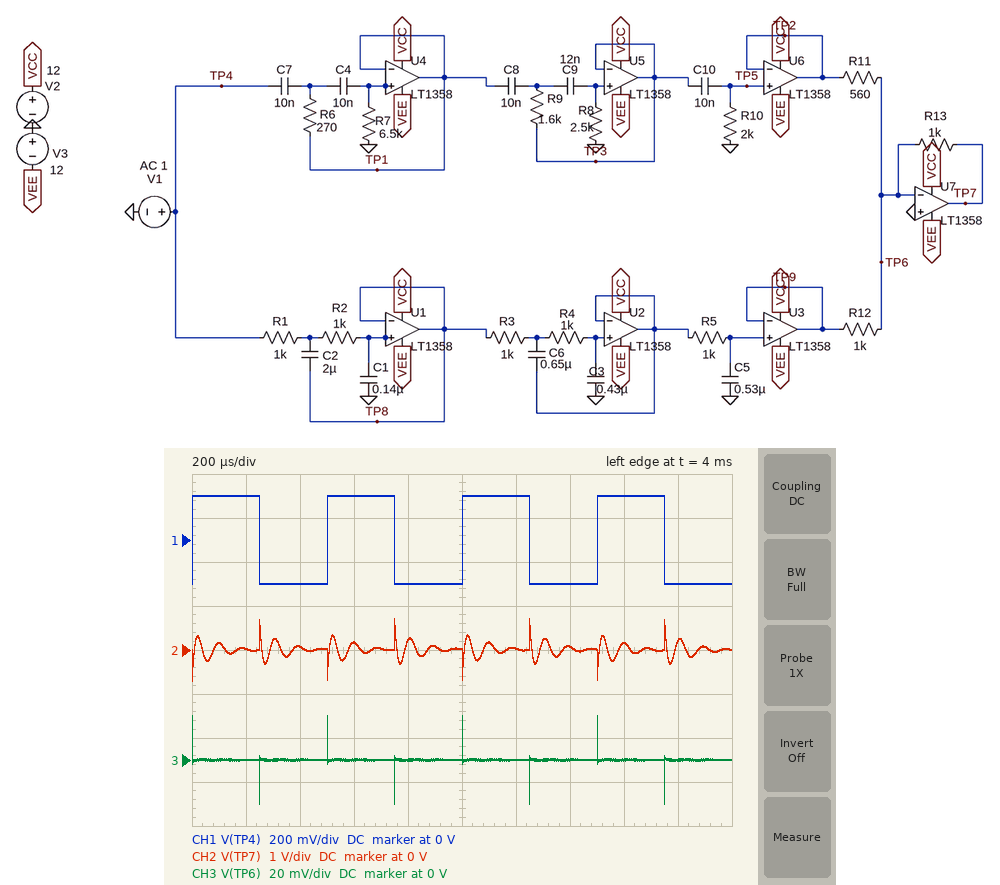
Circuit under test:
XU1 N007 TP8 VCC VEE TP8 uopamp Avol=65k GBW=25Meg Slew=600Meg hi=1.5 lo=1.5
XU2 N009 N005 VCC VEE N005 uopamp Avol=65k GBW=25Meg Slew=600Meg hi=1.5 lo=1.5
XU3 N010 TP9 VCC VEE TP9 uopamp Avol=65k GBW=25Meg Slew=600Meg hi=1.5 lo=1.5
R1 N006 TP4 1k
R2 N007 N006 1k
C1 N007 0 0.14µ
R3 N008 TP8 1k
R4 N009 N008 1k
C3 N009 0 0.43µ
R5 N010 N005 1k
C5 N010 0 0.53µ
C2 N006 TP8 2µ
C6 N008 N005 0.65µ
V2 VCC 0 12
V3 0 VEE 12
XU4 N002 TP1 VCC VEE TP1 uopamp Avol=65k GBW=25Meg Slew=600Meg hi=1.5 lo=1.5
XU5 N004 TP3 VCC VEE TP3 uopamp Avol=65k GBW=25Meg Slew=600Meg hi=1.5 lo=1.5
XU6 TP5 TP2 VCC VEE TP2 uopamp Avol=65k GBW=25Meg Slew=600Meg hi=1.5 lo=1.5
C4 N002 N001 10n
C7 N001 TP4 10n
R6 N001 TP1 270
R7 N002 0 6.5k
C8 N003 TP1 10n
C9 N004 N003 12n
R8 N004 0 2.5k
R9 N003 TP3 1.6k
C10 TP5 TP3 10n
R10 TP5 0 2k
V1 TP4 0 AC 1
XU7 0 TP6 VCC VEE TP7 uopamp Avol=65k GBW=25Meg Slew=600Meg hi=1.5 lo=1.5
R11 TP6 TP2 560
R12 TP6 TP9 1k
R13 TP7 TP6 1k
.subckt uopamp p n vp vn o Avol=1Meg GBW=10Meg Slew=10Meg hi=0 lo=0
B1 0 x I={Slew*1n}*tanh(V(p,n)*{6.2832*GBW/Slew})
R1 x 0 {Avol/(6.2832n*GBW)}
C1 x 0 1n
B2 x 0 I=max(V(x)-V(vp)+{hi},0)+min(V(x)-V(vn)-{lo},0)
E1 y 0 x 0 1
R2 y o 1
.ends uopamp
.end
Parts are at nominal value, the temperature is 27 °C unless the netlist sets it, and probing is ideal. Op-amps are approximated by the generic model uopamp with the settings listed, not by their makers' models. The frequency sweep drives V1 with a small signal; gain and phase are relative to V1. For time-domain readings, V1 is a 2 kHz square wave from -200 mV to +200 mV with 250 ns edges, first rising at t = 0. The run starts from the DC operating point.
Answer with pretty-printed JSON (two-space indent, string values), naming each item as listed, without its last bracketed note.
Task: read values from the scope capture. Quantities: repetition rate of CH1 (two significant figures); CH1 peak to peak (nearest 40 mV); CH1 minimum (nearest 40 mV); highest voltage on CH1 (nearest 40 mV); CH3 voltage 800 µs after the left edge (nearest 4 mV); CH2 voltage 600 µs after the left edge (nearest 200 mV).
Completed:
{
  "repetition rate of CH1": "2.0 kHz",
  "CH1 peak to peak": "400 mV",
  "CH1 minimum": "-200 mV",
  "highest voltage on CH1": "200 mV",
  "CH3 voltage 800 µs after the left edge": "0 V",
  "CH2 voltage 600 µs after the left edge": "200 mV"
}
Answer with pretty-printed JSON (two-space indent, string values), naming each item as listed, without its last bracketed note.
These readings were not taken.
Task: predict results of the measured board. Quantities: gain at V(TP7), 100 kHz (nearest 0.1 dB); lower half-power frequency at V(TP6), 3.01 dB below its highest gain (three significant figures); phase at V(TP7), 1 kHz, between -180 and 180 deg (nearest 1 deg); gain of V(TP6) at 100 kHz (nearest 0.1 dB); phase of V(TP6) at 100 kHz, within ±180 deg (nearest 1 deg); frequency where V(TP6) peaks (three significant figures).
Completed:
{
  "gain at V(TP7), 100 kHz": "5.1 dB",
  "lower half-power frequency at V(TP6), 3.01 dB below its highest gain": "3.72 MHz",
  "phase at V(TP7), 1 kHz, between -180 and 180 deg": "146 deg",
  "gain of V(TP6) at 100 kHz": "-42.9 dB",
  "phase of V(TP6) at 100 kHz, within ±180 deg": "102 deg",
  "frequency where V(TP6) peaks": "9.04 MHz"
}
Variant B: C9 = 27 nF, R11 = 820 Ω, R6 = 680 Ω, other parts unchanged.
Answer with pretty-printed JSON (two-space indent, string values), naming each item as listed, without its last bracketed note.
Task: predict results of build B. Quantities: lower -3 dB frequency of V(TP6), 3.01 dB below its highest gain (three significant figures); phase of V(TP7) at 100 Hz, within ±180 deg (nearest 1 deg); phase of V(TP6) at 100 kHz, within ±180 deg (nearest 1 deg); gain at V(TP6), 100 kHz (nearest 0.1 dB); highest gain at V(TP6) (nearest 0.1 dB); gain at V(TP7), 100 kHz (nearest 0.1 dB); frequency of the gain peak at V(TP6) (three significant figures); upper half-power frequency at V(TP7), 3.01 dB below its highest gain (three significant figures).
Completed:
{
  "lower -3 dB frequency of V(TP6), 3.01 dB below its highest gain": "4.08 MHz",
  "phase of V(TP7) at 100 Hz, within ±180 deg": "119 deg",
  "phase of V(TP6) at 100 kHz, within ±180 deg": "101 deg",
  "gain at V(TP6), 100 kHz": "-46.2 dB",
  "highest gain at V(TP6)": "-12.4 dB",
  "gain at V(TP7), 100 kHz": "1.7 dB",
  "frequency of the gain peak at V(TP6)": "9.68 MHz",
  "upper half-power frequency at V(TP7), 3.01 dB below its highest gain": "5.87 MHz"
}
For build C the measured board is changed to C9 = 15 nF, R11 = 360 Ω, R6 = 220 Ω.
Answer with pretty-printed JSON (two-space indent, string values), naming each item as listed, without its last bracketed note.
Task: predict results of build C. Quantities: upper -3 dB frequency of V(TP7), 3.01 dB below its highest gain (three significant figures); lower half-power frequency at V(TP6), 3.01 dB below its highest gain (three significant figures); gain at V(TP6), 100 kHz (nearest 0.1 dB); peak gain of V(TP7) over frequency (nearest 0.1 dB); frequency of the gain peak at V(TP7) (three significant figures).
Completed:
{
  "upper -3 dB frequency of V(TP7), 3.01 dB below its highest gain": "18.9 kHz",
  "lower half-power frequency at V(TP6), 3.01 dB below its highest gain": "3.22 MHz",
  "gain at V(TP6), 100 kHz": "-39.0 dB",
  "peak gain of V(TP7) over frequency": "15.7 dB",
  "frequency of the gain peak at V(TP7)": "14.0 kHz"
}
